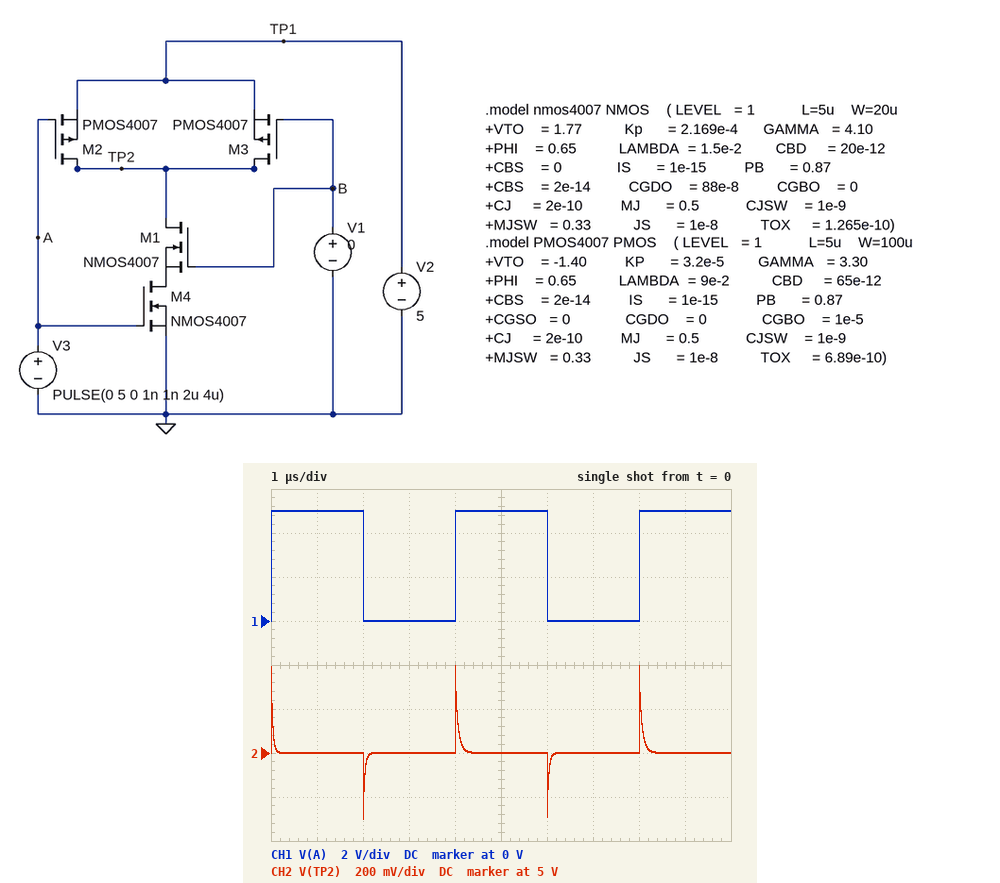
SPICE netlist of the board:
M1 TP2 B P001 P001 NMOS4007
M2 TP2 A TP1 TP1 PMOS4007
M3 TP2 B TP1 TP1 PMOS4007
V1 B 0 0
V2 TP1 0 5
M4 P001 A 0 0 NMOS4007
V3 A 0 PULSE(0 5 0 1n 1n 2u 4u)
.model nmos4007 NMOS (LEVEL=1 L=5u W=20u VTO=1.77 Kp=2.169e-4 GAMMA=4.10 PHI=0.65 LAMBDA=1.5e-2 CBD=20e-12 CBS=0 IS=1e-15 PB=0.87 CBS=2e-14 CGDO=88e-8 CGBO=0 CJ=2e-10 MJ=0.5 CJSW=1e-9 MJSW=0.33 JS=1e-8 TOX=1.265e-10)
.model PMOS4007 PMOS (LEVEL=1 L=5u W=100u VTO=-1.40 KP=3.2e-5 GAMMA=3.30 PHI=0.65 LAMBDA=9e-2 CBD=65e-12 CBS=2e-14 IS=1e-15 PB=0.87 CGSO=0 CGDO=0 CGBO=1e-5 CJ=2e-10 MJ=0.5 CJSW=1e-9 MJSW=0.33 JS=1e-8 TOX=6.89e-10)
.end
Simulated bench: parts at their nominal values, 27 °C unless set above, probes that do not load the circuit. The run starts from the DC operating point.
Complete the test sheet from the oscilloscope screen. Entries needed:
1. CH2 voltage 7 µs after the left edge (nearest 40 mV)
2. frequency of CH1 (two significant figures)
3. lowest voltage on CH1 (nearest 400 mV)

5.00 V
250 kHz
0 V
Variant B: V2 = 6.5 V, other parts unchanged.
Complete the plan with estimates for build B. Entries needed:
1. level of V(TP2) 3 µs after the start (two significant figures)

6.5 V
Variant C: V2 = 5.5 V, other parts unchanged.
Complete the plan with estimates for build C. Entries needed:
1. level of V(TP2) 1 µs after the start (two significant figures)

5.5 V
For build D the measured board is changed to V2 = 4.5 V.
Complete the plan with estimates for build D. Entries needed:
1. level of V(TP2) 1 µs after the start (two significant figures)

4.5 V
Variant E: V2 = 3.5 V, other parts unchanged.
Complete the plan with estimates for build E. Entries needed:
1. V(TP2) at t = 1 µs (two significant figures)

3.5 V
